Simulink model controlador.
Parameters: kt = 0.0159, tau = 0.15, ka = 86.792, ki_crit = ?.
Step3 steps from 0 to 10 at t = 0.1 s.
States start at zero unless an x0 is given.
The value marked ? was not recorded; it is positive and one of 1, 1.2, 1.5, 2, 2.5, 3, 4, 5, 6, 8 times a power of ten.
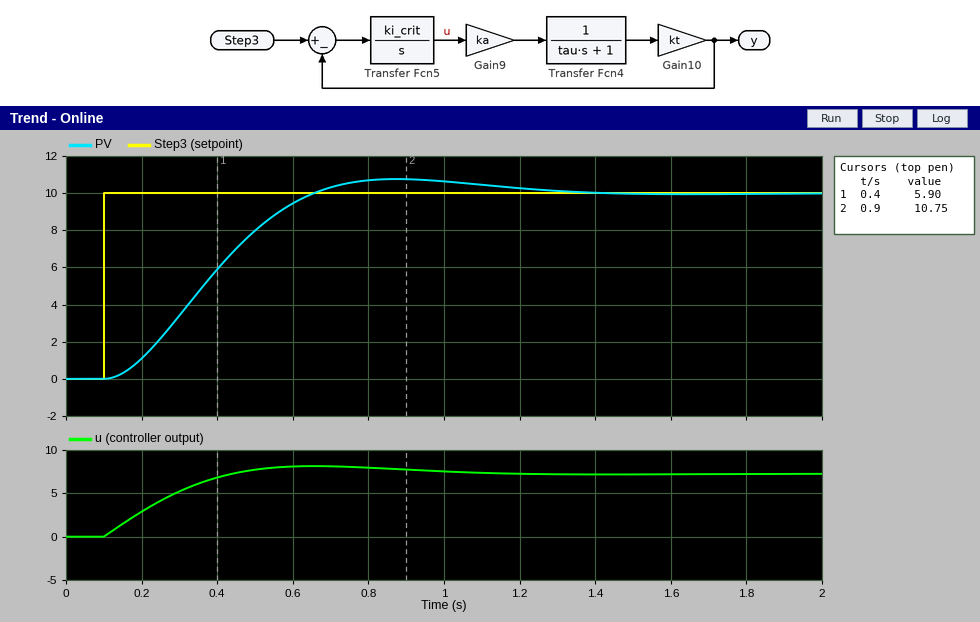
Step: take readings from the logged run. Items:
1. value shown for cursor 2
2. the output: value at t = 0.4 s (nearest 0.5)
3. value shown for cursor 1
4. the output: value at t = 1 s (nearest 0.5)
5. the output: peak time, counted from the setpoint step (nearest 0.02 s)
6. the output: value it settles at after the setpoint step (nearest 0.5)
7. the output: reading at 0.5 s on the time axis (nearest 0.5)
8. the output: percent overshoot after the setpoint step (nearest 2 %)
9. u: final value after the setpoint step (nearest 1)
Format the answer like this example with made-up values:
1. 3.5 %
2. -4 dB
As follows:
1. 10.75
2. 6.0
3. 5.90
4. 10.5
5. 0.78 s
6. 10.0
7. 8.0
8. 8 %
9. 7
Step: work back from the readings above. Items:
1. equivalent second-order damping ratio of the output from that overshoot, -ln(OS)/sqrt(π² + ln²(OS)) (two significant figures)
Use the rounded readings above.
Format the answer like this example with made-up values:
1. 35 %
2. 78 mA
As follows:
1. 0.63
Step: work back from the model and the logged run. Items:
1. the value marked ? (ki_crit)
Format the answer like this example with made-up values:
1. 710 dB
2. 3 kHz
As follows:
1. 3
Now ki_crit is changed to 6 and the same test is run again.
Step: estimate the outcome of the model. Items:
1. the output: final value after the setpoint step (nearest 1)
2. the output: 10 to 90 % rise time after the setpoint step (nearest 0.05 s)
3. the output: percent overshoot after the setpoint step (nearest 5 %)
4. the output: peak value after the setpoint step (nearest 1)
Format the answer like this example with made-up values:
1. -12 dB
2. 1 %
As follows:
1. 10
2. 0.20 s
3. 20 %
4. 12
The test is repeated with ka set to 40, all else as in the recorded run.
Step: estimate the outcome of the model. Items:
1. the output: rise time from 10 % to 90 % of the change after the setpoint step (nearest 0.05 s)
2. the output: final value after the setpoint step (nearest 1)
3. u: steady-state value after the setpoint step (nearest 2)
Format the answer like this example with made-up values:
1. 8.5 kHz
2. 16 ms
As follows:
1. 0.85 s
2. 10
3. 16
